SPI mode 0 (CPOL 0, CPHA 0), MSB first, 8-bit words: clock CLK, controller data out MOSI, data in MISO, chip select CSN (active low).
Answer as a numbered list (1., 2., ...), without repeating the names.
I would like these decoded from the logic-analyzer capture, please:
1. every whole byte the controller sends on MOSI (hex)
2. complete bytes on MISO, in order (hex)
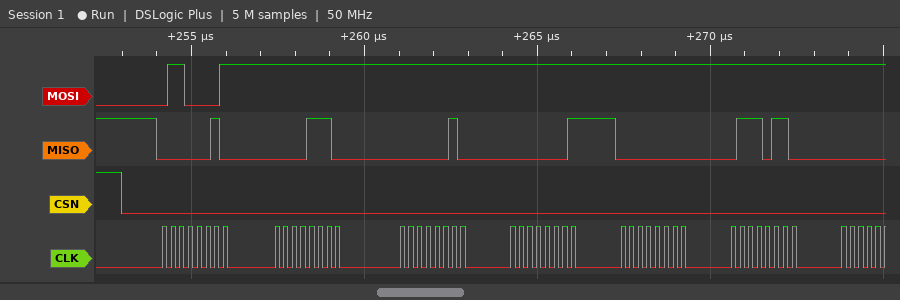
1. 61 FF FF FF FF FF
2. 02 0E 02 01 00 76
